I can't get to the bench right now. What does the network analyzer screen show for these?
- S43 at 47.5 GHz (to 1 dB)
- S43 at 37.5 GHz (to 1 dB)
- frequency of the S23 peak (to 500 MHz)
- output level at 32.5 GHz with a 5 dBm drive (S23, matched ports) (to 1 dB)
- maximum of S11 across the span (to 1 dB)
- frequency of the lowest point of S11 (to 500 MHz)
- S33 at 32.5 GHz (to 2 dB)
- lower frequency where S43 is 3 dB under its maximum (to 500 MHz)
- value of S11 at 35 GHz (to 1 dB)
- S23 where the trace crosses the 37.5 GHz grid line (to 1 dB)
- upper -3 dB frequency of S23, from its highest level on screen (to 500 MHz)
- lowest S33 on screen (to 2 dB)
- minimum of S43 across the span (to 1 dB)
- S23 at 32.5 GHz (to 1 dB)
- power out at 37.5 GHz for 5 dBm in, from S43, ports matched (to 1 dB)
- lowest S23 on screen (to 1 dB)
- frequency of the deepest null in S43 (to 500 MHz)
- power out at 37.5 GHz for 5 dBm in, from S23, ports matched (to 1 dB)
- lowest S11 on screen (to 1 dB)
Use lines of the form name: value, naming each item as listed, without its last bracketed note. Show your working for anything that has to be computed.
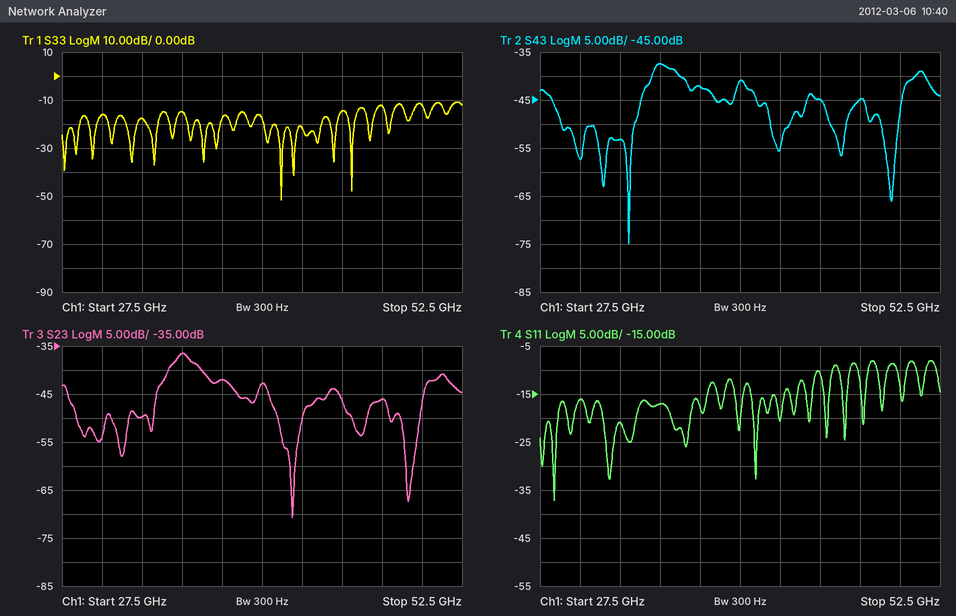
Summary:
S43 at 47.5 GHz: -45 dB
S43 at 37.5 GHz: -42 dB
frequency of the S23 peak: 35.0 GHz
output level at 32.5 GHz with a 5 dBm drive (S23, matched ports): 5 dBm + (-50 dB) = -45 dBm
maximum of S11 across the span: -8 dB
frequency of the lowest point of S11: 28.5 GHz
S33 at 32.5 GHz: -18 dB
lower frequency where S43 is 3 dB under its maximum: 34.5 GHz
value of S11 at 35 GHz: -17 dB
S23 where the trace crosses the 37.5 GHz grid line: -42 dB
upper -3 dB frequency of S23, from its highest level on screen: 36.0 GHz
lowest S33 on screen: -52 dB
minimum of S43 across the span: -75 dB
S23 at 32.5 GHz: -50 dB
power out at 37.5 GHz for 5 dBm in, from S43, ports matched: 5 dBm + (-42 dB) = -37 dBm
lowest S23 on screen: -71 dB
frequency of the deepest null in S43: 33.0 GHz
power out at 37.5 GHz for 5 dBm in, from S23, ports matched: 5 dBm + (-42 dB) = -37 dBm
lowest S11 on screen: -37 dB
